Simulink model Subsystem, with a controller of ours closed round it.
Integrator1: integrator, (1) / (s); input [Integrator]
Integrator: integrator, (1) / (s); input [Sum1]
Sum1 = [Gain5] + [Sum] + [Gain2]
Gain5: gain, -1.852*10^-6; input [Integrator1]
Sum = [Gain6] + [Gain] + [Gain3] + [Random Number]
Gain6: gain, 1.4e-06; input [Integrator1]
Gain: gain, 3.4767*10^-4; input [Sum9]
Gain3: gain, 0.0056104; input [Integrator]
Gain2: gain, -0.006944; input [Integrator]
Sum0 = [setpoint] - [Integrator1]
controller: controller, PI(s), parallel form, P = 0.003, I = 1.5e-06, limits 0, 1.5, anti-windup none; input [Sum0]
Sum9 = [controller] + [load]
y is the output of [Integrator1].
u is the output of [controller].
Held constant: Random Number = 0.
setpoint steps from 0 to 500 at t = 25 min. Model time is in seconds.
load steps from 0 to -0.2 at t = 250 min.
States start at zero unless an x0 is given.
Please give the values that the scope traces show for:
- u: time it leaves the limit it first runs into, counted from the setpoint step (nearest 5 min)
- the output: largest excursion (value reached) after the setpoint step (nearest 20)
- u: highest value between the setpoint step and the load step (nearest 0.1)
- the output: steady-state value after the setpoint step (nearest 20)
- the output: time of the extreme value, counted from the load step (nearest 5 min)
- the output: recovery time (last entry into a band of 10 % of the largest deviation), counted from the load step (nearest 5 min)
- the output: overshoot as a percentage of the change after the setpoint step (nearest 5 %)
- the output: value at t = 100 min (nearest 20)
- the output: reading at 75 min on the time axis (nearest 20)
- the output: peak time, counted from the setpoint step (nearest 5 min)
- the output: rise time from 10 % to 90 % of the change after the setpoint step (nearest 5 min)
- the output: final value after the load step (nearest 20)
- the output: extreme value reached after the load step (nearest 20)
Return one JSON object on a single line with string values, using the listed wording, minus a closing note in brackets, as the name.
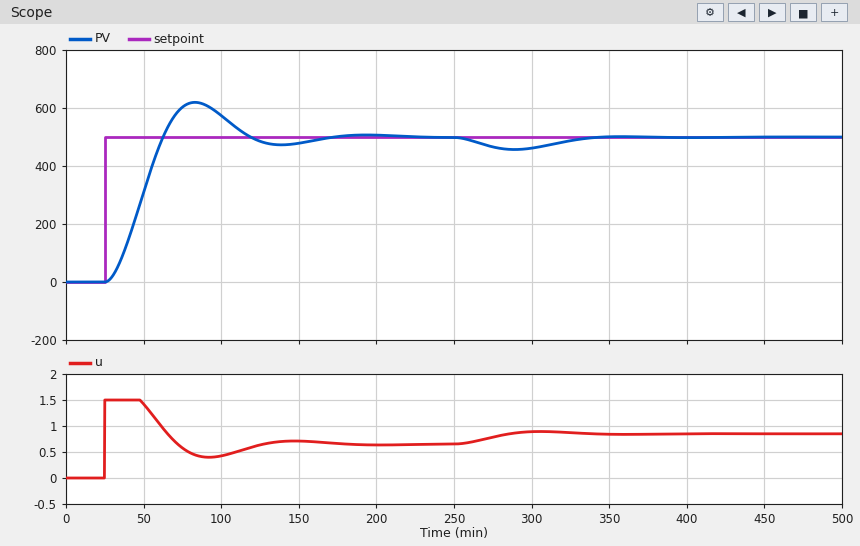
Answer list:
{"u: time it leaves the limit it first runs into, counted from the setpoint step": "25 min", "the output: largest excursion (value reached) after the setpoint step": "620", "u: highest value between the setpoint step and the load step": "1.5", "the output: steady-state value after the setpoint step": "500", "the output: time of the extreme value, counted from the load step": "40 min", "the output: recovery time (last entry into a band of 10 % of the largest deviation), counted from the load step": "85 min", "the output: overshoot as a percentage of the change after the setpoint step": "25 %", "the output: value at t = 100 min": "580", "the output: reading at 75 min on the time axis": "600", "the output: peak time, counted from the setpoint step": "60 min", "the output: rise time from 10 % to 90 % of the change after the setpoint step": "25 min", "the output: final value after the load step": "500", "the output: extreme value reached after the load step": "460"}
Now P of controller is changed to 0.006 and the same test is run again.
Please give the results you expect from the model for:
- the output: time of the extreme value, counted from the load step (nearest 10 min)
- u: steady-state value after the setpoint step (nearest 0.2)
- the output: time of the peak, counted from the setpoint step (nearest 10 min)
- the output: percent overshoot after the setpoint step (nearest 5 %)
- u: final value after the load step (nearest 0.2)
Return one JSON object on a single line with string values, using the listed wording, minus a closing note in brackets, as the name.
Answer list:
{"the output: time of the extreme value, counted from the load step": "30 min", "u: steady-state value after the setpoint step": "0.6", "the output: time of the peak, counted from the setpoint step": "50 min", "the output: percent overshoot after the setpoint step": "20 %", "u: final value after the load step": "0.8"}
